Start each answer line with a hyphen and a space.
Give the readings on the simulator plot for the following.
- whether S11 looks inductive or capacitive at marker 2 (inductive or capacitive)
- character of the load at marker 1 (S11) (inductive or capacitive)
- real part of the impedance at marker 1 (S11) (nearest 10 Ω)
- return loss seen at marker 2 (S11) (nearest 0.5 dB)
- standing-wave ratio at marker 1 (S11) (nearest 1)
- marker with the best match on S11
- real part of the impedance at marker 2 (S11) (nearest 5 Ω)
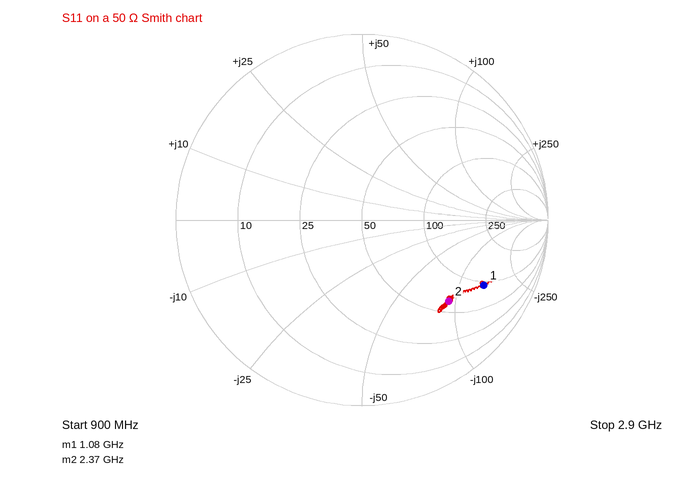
- capacitive
- capacitive
- 90 Ω
- 4.0 dB
- 7
- marker 2
- 60 Ω
